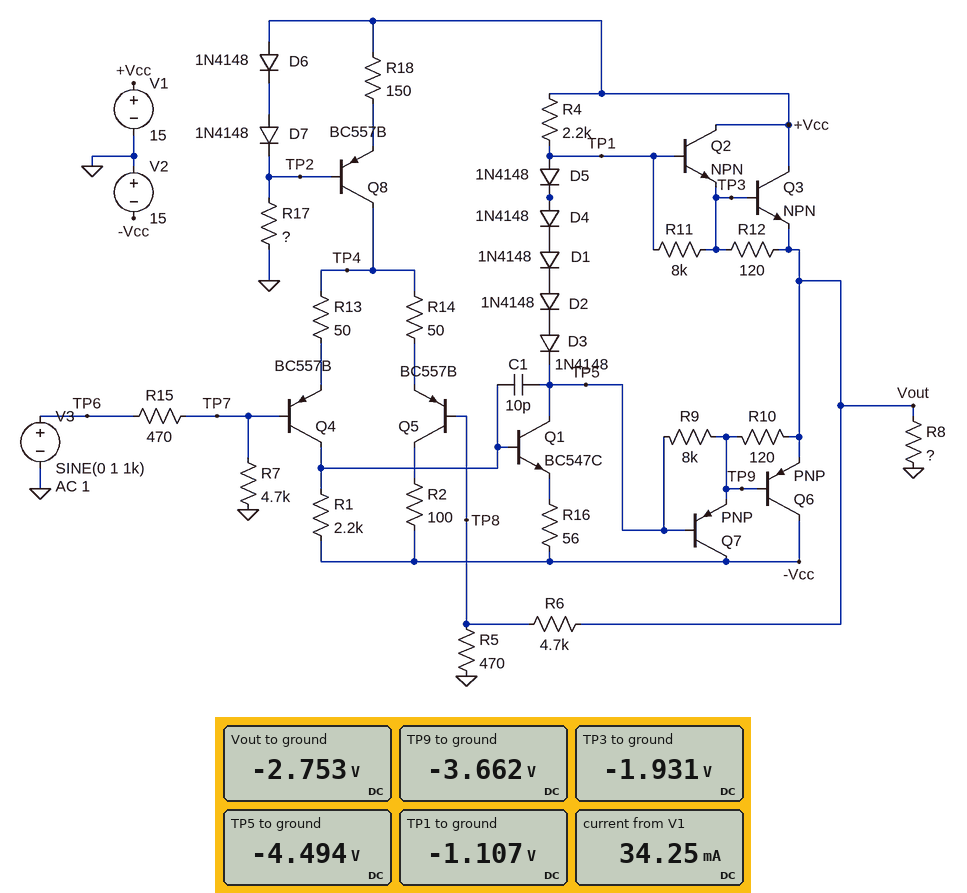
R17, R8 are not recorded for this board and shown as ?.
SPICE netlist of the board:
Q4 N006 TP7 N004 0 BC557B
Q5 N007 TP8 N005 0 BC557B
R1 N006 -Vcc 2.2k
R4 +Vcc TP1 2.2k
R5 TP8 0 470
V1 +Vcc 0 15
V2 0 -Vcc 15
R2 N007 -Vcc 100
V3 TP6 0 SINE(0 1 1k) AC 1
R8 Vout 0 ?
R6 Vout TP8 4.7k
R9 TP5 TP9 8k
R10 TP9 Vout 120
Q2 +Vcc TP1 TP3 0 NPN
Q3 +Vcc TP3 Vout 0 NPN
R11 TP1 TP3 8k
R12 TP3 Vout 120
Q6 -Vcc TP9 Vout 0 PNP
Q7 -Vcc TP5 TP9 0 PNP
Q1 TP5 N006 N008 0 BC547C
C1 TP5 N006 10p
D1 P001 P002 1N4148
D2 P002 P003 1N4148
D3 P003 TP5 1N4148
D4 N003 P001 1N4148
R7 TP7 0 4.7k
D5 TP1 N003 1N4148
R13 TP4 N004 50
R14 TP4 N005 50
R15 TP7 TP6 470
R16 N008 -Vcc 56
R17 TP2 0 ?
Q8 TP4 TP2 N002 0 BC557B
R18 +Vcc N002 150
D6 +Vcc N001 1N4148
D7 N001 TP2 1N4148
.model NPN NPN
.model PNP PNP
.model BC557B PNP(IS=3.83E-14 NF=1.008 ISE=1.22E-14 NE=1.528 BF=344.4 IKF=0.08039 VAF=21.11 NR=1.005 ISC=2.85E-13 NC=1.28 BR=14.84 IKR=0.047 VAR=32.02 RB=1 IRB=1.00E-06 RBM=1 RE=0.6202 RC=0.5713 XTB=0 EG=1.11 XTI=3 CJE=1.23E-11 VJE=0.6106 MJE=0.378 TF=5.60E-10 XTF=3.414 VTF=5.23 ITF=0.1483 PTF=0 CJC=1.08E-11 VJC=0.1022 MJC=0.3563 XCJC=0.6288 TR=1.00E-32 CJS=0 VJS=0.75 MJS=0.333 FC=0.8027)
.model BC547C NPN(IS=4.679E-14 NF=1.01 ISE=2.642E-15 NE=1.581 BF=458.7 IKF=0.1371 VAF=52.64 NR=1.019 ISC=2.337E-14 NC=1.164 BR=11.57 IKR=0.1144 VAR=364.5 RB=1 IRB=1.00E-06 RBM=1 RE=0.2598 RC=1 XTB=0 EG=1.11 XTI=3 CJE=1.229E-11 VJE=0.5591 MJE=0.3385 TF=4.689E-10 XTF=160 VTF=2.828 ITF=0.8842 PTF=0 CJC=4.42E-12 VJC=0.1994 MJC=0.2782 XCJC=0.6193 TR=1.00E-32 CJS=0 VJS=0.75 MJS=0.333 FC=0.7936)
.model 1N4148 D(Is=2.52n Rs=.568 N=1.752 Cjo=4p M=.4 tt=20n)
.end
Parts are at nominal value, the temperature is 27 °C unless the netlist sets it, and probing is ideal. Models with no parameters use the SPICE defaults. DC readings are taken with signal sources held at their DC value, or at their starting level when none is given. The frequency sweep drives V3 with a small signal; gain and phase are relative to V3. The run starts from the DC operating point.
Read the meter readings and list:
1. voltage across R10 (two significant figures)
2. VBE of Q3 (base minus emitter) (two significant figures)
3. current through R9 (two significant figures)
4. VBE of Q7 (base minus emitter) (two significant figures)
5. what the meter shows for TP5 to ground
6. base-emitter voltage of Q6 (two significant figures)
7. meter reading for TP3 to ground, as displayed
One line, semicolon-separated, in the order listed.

910 mV; 820 mV; 100 µA; -830 mV; -4.494 V; -910 mV; -1.931 V
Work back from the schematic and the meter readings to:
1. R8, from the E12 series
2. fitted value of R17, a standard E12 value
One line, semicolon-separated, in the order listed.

15 Ω; 1.5 kΩ
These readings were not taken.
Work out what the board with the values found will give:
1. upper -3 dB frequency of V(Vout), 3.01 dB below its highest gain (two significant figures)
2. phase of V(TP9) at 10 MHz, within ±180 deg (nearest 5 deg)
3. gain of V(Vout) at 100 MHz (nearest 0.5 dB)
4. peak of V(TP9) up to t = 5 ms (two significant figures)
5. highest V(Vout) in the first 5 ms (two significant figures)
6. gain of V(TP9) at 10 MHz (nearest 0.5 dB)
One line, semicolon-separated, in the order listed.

11 MHz; -95 deg; -15.5 dB; 6.4 V; 7.0 V; 17.5 dB
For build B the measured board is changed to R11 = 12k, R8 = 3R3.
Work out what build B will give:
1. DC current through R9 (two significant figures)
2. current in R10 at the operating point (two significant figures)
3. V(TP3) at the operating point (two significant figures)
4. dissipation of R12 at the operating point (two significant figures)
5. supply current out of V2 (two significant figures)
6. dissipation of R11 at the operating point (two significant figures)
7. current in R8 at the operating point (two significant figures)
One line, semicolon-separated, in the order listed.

110 µA; 7.9 mA; -2.0 V; 5.0 mW; 850 mA; 56 µW; 830 mA
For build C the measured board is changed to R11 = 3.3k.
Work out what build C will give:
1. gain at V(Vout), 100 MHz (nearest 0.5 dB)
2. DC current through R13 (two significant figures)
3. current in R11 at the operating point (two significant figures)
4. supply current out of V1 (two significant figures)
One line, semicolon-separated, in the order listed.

-15.5 dB; 500 µA; 250 µA; 33 mA
